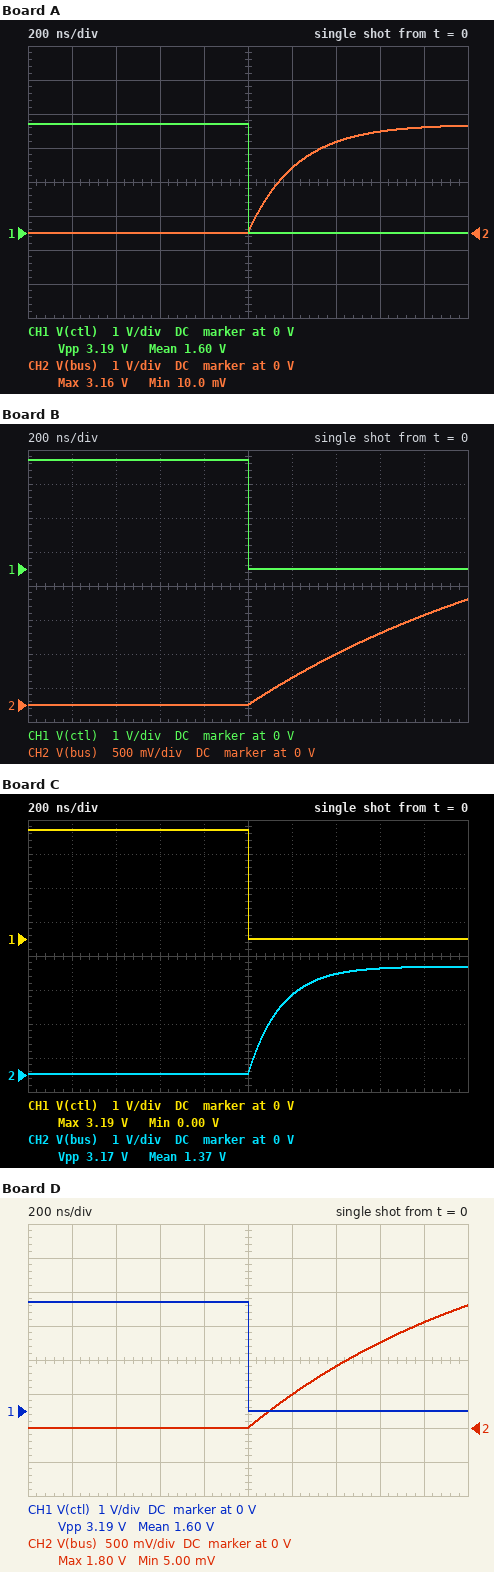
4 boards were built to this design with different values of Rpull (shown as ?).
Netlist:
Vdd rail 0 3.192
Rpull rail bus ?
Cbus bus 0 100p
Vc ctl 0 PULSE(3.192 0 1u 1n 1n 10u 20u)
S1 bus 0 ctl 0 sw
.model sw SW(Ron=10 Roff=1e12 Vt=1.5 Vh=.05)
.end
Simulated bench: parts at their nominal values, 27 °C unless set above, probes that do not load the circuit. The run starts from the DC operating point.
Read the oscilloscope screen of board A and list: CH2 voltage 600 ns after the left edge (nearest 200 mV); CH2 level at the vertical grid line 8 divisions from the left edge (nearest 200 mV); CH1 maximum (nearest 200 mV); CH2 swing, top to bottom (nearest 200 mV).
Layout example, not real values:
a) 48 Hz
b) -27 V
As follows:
a) 0 V
b) 3.0 V
c) 3.2 V
d) 3.2 V
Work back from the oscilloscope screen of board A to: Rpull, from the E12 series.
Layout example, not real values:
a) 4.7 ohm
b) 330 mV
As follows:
a) 2.2 kΩ
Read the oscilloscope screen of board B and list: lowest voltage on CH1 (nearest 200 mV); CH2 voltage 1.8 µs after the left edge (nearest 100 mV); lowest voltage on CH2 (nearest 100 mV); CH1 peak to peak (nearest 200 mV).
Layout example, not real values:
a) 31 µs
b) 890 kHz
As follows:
a) 0 V
b) 1.3 V
c) 0 V
d) 3.2 V
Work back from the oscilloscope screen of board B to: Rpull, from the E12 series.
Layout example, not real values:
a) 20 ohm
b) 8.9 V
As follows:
a) 15 kΩ
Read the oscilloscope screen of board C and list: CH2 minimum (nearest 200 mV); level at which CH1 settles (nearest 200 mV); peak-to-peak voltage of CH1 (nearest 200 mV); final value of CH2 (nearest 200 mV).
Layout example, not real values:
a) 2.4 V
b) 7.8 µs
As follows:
a) 0 V
b) 0 V
c) 3.2 V
d) 3.2 V
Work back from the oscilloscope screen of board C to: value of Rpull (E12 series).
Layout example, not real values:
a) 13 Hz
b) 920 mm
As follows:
a) 1.5 kΩ
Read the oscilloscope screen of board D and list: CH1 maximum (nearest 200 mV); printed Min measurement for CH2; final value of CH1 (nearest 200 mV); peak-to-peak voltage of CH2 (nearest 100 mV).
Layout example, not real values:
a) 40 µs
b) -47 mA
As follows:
a) 3.2 V
b) 5.00 mV
c) 0 V
d) 1.8 V
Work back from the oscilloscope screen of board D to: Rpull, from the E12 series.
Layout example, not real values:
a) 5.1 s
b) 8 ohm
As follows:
a) 12 kΩ
